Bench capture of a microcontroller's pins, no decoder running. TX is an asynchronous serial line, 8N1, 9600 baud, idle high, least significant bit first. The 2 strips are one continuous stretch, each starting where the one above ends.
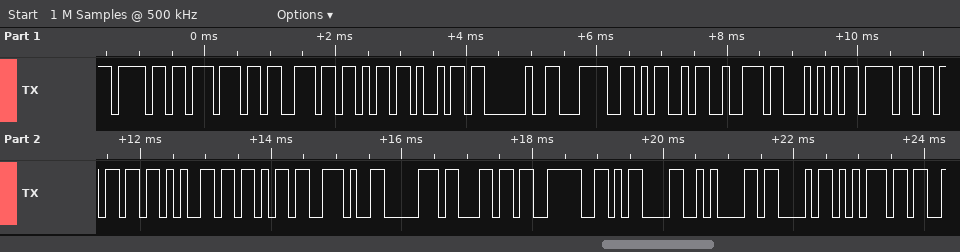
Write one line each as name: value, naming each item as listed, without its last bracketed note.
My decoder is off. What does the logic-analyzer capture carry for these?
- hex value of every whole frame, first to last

hex value of every whole frame, first to last: 0x6F 0x77 0x73 0x6B 0x69 0x20 0x3C 0x4D 0x72 0x54 0x6F 0x6D 0x65 0x6B 0x2E 0x70 0x6C 0x3E 0x0D 0x0A 0x43 0x75
